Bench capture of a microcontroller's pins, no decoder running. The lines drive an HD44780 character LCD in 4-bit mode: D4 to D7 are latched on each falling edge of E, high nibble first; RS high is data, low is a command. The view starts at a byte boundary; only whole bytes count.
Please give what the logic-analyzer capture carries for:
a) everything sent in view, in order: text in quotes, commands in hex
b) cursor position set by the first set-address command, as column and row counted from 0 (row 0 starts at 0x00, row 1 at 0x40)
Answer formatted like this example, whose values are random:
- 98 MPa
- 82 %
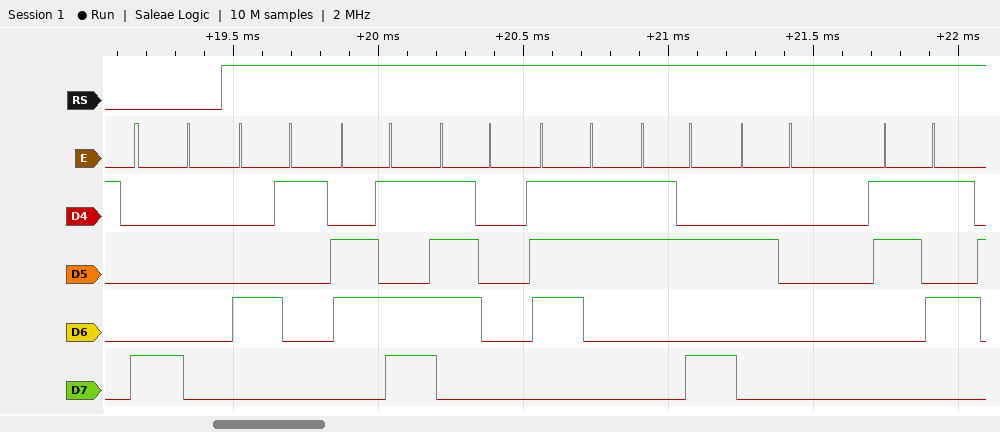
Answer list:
- 0x80 "Amps: 5"
- column 0, row 0
